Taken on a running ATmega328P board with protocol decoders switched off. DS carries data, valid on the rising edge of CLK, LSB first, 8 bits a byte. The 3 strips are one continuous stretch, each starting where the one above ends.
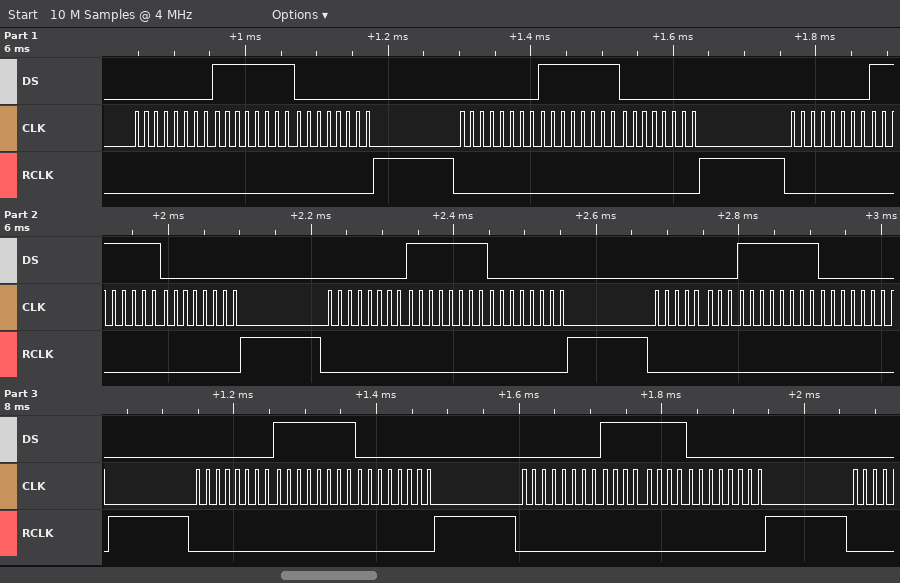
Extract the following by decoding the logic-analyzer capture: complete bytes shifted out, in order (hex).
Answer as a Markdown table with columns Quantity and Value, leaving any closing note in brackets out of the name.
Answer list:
| Quantity | Value |
|---|---|
| complete bytes shifted out, in order | 00 FF 00 00 FF 00 00 FF 00 00 FF 00 00 FF 00 00 FF 00 00 FF 00 |
